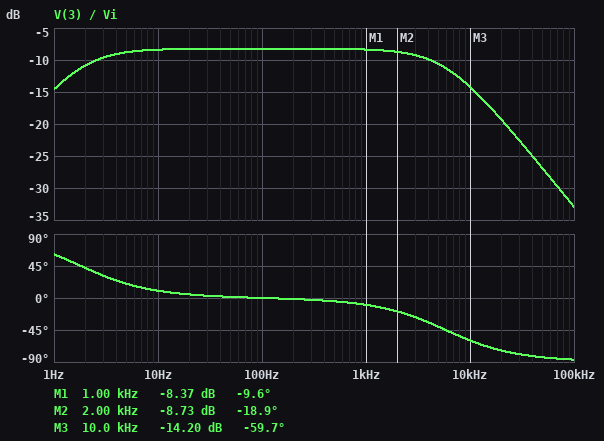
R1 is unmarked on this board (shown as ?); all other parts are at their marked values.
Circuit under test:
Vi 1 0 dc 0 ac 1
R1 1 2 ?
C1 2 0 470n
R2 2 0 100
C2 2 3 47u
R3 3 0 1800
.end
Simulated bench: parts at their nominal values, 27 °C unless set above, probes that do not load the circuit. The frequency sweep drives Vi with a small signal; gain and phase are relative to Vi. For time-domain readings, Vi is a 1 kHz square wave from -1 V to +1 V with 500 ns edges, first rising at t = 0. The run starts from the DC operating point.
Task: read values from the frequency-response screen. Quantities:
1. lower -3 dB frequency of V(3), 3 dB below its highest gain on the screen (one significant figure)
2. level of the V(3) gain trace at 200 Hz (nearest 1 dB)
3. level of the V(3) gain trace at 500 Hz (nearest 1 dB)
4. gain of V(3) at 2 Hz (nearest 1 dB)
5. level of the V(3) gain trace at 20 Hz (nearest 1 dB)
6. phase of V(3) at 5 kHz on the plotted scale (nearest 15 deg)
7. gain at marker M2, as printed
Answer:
2 Hz
-8 dB
-8 dB
-11 dB
-8 dB
-45 deg
-8.73 dB
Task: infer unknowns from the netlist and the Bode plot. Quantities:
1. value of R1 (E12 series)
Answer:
150 Ω
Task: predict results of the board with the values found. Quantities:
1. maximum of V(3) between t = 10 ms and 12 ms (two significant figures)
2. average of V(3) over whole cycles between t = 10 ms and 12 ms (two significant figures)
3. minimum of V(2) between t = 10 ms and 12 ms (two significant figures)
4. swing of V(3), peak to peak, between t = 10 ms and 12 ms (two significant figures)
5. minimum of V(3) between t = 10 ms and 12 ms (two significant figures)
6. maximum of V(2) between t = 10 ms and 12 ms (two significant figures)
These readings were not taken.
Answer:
730 mV
340 mV
-400 mV
780 mV
-50 mV
380 mV
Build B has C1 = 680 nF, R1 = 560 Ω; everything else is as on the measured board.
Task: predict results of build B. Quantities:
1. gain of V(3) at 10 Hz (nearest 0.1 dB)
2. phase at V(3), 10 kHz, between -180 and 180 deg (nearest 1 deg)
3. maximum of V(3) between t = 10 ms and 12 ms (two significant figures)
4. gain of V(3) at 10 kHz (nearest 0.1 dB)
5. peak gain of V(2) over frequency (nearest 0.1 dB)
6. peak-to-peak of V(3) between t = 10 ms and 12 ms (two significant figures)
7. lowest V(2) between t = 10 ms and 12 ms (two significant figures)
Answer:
-16.9 dB
-74 deg
270 mV
-27.9 dB
-16.4 dB
290 mV
-150 mV
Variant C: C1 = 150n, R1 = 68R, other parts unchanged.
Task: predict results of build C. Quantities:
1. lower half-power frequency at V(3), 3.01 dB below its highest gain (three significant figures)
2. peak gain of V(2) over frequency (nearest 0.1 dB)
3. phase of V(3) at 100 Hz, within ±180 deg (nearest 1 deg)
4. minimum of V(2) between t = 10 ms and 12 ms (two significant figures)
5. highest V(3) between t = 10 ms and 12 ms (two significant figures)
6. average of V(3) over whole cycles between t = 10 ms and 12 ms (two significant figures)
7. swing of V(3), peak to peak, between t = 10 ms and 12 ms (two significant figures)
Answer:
1.84 Hz
-4.5 dB
1 deg
-590 mV
1.1 V
510 mV
1.2 V
